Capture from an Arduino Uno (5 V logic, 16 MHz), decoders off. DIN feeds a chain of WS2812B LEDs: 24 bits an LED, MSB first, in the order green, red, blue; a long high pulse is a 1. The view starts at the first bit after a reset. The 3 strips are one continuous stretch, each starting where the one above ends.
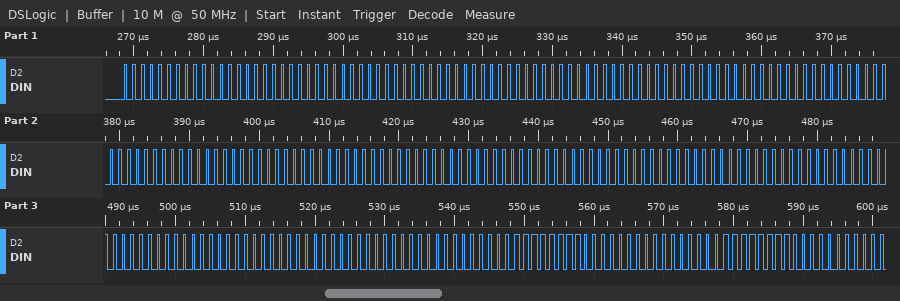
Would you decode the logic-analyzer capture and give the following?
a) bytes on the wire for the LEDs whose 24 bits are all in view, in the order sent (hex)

00 00 00 00 00 00 00 00 00 00 00 00 00 00 00 00 00 00 00 00 00 00 00 00 00 00 00 00 FF 00 00 FF 00
